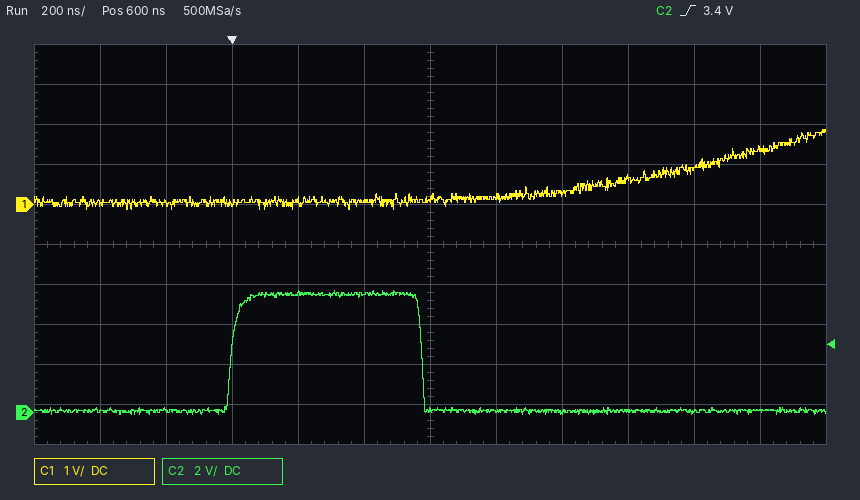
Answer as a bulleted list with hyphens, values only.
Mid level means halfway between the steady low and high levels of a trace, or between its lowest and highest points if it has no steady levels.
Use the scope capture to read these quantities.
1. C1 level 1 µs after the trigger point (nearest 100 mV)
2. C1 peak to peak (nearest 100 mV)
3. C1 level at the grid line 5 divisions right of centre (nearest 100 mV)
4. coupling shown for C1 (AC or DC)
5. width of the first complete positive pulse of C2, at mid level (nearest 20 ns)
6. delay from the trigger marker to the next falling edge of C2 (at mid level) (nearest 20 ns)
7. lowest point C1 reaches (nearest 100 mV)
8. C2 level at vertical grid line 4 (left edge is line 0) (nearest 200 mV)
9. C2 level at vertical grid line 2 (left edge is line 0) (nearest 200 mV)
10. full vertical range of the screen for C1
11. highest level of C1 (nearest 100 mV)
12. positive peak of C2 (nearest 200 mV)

- 300 mV
- 2.0 V
- 1.4 V
- DC
- 580 ns
- 580 ns
- -100 mV
- 6.0 V
- 200 mV
- 10 V
- 1.9 V
- 6.0 V
